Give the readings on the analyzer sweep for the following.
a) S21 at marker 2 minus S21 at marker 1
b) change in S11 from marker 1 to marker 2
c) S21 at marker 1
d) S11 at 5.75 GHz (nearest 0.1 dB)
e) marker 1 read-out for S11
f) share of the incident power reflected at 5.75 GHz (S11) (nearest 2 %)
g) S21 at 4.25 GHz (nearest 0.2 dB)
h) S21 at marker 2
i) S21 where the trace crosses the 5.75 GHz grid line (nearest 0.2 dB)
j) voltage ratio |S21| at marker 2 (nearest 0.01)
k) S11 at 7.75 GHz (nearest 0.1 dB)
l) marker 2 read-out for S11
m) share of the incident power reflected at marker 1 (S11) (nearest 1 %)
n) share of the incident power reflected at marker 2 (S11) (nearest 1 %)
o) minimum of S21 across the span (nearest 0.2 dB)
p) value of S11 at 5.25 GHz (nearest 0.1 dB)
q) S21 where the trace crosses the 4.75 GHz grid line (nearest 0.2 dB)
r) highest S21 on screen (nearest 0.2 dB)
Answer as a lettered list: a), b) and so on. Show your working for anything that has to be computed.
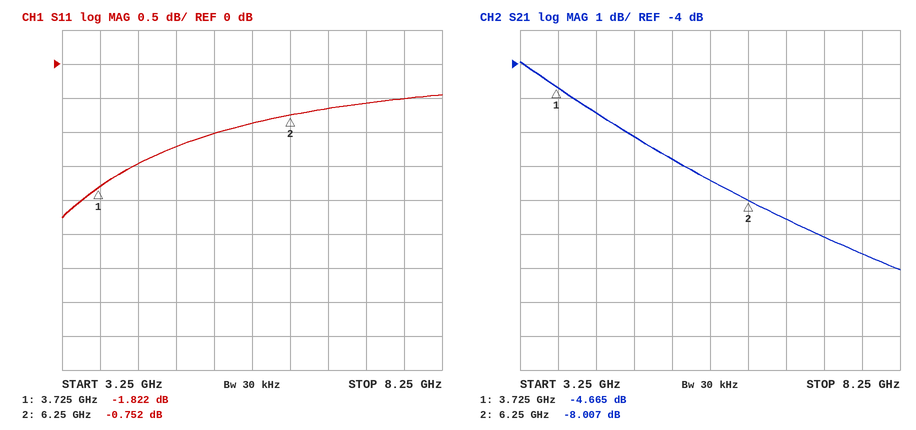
a) -8.007 − (-4.665) = -3.342 dB
b) -0.752 − (-1.822) = 1.070 dB
c) -4.665 dB
d) -0.9 dB
e) -1.822 dB
f) 10^(-0.9/10) ≈ 81.3 %, so 82 % to the nearest 2 %
g) -5.4 dB
h) -8.007 dB
i) -7.4 dB
j) 10^(-8.007/20) ≈ 0.40
k) -0.5 dB
l) -0.752 dB
m) 10^(-1.822/10) ≈ 66 %
n) 10^(-0.752/10) ≈ 84 %
o) -10.0 dB
p) -1.0 dB
q) -6.2 dB
r) -4.0 dB
